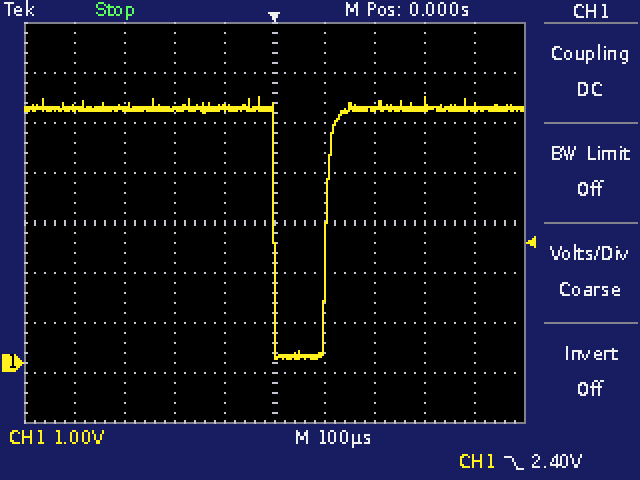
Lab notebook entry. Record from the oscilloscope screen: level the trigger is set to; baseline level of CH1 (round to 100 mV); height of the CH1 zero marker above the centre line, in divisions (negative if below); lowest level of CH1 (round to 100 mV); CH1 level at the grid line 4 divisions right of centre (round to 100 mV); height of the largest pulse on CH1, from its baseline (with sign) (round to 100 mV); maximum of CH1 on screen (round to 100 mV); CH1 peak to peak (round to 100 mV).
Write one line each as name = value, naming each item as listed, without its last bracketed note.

level the trigger is set to = 2.40 V
baseline level of CH1 = 5.1 V
height of the CH1 zero marker above the centre line, in divisions = -2.8 div
lowest level of CH1 = 100 mV
CH1 level at the grid line 4 divisions right of centre = 5.1 V
height of the largest pulse on CH1, from its baseline (with sign) = -5.0 V
maximum of CH1 on screen = 5.3 V
CH1 peak to peak = 5.2 V
